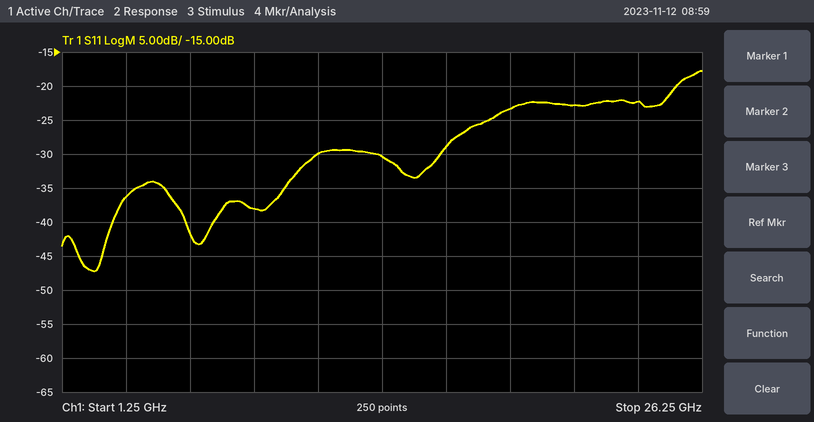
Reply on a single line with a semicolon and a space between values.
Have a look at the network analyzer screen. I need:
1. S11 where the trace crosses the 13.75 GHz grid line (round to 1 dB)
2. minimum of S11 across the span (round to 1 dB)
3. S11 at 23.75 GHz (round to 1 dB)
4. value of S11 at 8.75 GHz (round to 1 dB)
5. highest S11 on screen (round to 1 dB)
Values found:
-30 dB; -47 dB; -22 dB; -38 dB; -18 dB
